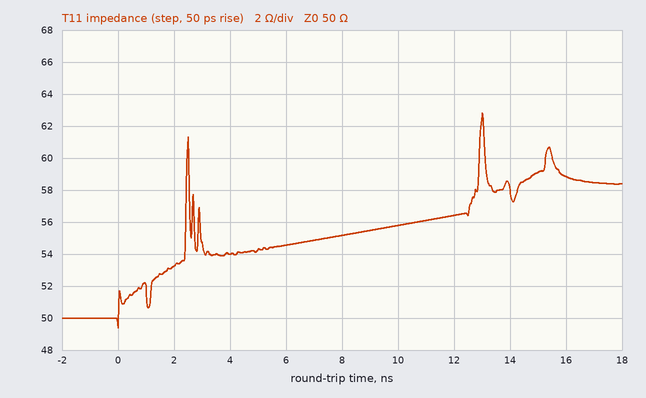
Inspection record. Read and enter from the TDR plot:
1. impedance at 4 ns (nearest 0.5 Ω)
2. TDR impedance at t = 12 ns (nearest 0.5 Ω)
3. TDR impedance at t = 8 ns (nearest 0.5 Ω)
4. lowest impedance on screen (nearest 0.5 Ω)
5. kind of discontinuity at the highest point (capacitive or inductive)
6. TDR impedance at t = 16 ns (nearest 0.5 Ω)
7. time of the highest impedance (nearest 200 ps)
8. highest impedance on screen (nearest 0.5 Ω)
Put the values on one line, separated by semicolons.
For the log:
54.0 Ω; 56.5 Ω; 55.0 Ω; 49.5 Ω; inductive; 59.0 Ω; 13.0 ns; 63.0 Ω
